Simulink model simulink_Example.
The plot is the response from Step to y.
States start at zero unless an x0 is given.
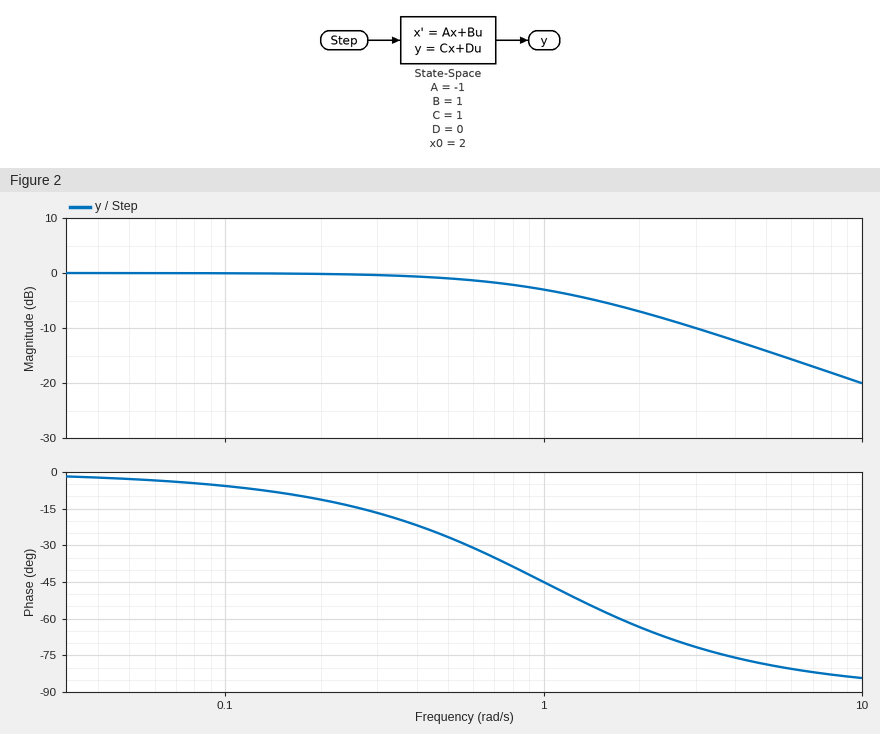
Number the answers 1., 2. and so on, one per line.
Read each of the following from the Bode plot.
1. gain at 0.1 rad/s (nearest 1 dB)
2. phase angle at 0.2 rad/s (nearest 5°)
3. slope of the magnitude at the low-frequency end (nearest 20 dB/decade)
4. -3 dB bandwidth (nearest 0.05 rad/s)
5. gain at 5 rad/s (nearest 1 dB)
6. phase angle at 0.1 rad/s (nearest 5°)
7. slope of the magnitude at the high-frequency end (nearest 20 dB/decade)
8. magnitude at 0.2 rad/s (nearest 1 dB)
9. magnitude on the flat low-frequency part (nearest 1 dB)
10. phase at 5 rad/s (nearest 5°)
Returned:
1. 0 dB
2. -10°
3. 0 dB/decade
4. 1.00 rad/s
5. -14 dB
6. -5°
7. -20 dB/decade
8. 0 dB
9. 0 dB
10. -80°
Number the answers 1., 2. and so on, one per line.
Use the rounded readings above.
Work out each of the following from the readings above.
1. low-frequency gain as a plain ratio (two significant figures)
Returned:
1. 1.0
